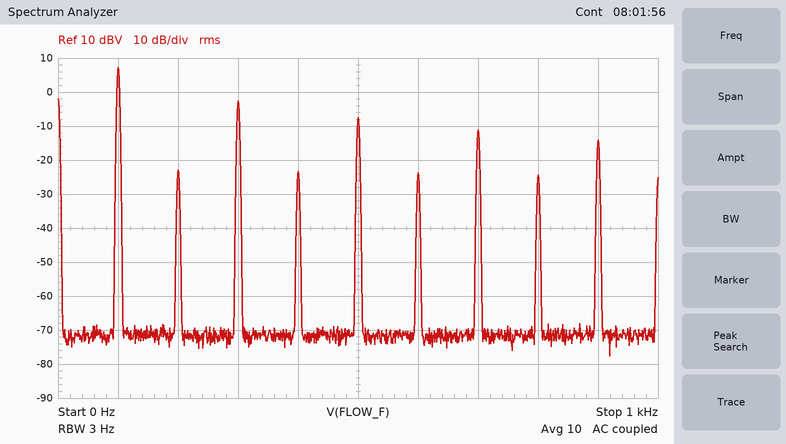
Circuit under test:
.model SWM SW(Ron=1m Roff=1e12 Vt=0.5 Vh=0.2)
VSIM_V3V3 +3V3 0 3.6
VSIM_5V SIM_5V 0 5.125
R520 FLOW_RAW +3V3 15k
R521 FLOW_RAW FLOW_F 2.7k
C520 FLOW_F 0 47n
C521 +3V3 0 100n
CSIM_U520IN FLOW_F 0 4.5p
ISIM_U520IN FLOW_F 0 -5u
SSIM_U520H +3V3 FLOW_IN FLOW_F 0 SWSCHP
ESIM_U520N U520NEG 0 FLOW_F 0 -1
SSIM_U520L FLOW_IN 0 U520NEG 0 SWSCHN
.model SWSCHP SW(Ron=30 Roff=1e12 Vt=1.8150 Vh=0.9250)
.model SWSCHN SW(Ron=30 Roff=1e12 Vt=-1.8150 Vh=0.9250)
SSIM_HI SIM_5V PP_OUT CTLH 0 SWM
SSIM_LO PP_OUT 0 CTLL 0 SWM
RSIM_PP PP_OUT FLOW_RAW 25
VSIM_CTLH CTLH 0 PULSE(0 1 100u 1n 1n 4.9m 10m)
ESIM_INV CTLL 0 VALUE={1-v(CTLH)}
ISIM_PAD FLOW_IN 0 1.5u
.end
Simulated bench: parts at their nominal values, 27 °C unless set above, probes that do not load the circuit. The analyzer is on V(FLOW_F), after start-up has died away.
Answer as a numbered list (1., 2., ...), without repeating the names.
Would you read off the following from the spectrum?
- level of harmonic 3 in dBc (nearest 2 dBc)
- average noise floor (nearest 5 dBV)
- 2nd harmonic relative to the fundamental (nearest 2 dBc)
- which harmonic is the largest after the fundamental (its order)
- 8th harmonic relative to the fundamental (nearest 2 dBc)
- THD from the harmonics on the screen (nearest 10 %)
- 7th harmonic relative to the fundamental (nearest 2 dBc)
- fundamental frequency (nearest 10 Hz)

1. -10 dBc
2. -70 dBV
3. -30 dBc
4. 3
5. -32 dBc
6. 40 %
7. -18 dBc
8. 100 Hz
